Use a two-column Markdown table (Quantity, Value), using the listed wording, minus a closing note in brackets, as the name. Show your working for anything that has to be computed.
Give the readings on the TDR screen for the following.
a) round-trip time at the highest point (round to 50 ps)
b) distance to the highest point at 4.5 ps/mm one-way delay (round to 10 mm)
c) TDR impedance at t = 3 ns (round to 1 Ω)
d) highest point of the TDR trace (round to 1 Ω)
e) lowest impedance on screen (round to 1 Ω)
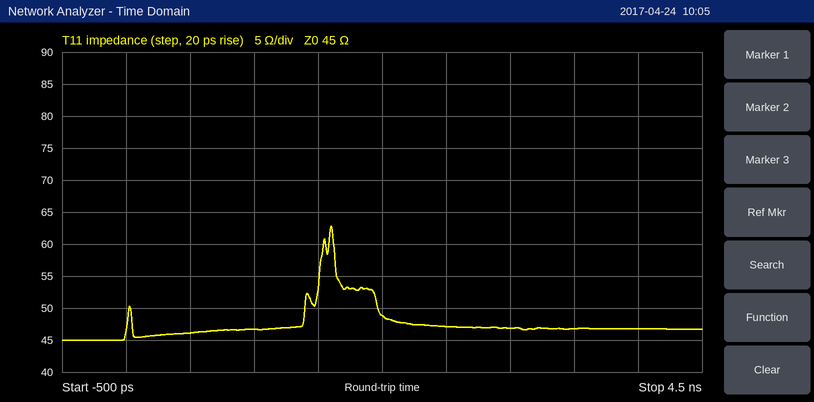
| Quantity | Value |
|---|---|
| round-trip time at the highest point | 1.60 ns |
| distance to the highest point at 4.5 ps/mm one-way delay | 1.60 ns / 2 / 4.5 ps/mm ≈ 178 mm, so 180 mm to the nearest 10 mm |
| TDR impedance at t = 3 ns | 47 Ω |
| highest point of the TDR trace | 63 Ω |
| lowest impedance on screen | 45 Ω |
